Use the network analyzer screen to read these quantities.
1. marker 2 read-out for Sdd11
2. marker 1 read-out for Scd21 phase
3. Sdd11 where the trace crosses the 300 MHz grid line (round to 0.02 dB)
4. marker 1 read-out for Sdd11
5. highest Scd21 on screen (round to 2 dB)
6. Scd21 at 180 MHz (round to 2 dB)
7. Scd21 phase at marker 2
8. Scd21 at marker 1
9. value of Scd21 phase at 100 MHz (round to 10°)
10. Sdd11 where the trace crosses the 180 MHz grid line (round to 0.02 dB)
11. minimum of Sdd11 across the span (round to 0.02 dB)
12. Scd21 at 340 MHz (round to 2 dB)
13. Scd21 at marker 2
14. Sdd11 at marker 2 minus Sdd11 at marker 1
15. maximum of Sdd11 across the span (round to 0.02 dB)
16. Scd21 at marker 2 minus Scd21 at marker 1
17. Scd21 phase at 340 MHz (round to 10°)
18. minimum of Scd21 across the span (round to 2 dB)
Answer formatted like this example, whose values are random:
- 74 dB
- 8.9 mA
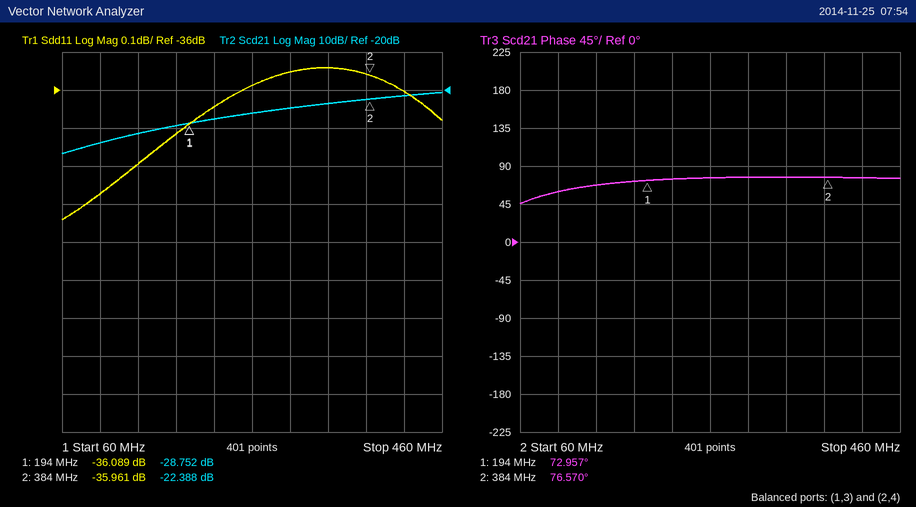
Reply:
- -35.961 dB
- 72.957°
- -35.96 dB
- -36.089 dB
- -20 dB
- -30 dB
- 76.570°
- -28.752 dB
- 60°
- -36.12 dB
- -36.34 dB
- -24 dB
- -22.388 dB
- 0.128 dB
- -35.94 dB
- 6.364 dB
- 80°
- -36 dB
